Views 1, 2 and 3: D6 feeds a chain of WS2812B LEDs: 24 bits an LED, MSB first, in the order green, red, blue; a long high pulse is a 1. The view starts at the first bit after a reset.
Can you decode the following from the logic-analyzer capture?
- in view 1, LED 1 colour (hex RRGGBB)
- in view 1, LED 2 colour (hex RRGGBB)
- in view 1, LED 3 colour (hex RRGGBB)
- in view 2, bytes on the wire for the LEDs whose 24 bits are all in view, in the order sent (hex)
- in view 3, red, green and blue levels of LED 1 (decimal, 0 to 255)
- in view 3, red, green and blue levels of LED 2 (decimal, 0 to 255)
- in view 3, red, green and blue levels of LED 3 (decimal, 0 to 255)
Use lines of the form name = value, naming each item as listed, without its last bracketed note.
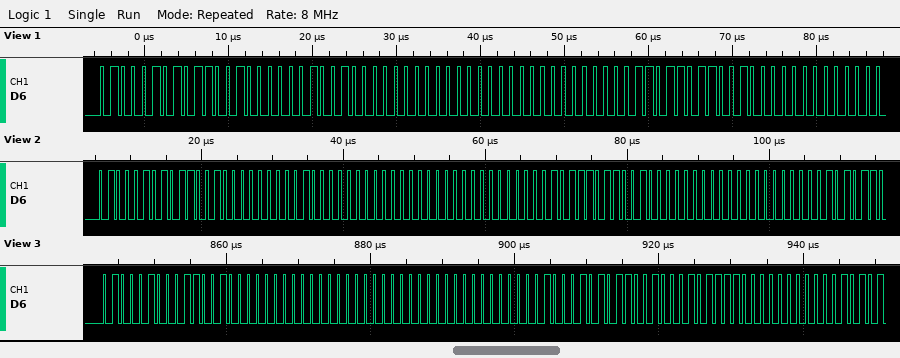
in view 1, LED 1 colour = #644509
in view 1, LED 2 colour = #000000
in view 1, LED 3 colour = #641B00
in view 2, bytes on the wire for the LEDs whose 24 bits are all in view, in the order sent = 45 64 01 00 00 00 17 64 00
in view 3, red, green and blue levels of LED 1 = 100, 68, 0
in view 3, red, green and blue levels of LED 2 = 0, 0, 0
in view 3, red, green and blue levels of LED 3 = 100, 69, 94
